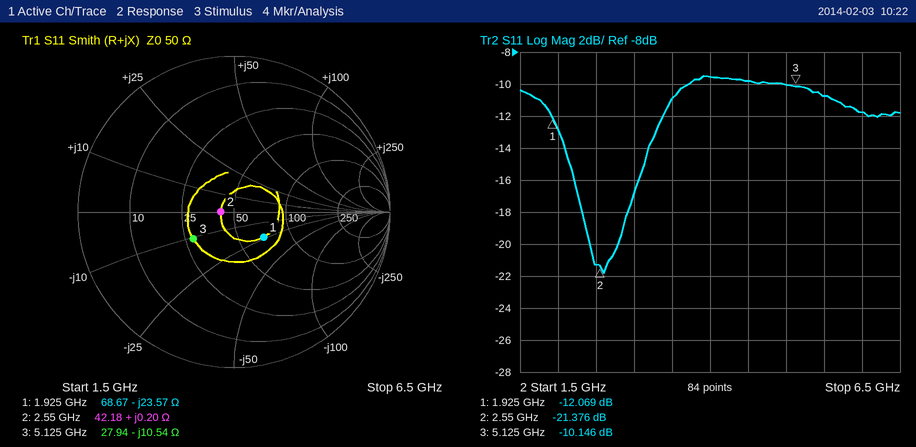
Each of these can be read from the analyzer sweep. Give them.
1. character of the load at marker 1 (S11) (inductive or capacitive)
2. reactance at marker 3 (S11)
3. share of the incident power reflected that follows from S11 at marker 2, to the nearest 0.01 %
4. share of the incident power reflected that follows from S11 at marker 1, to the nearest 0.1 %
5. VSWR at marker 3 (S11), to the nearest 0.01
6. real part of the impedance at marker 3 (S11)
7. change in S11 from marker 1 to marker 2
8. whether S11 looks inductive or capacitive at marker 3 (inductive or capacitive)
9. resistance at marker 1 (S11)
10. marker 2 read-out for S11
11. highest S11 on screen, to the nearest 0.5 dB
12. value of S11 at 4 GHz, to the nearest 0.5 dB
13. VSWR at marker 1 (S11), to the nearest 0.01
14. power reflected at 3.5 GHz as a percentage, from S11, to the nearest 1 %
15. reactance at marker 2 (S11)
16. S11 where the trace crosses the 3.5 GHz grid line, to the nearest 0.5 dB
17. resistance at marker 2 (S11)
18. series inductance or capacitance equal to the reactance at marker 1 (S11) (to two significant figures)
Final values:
capacitive
-10.54 Ω
0.73 %
6.2 %
1.90
27.94 Ω
-9.307 dB
capacitive
68.67 Ω
-21.376 dB
-9.5 dB
-9.5 dB
1.66
8 %
+0.20 Ω
-11.0 dB
42.18 Ω
3.5 pF
